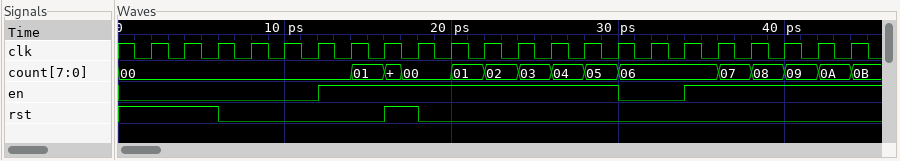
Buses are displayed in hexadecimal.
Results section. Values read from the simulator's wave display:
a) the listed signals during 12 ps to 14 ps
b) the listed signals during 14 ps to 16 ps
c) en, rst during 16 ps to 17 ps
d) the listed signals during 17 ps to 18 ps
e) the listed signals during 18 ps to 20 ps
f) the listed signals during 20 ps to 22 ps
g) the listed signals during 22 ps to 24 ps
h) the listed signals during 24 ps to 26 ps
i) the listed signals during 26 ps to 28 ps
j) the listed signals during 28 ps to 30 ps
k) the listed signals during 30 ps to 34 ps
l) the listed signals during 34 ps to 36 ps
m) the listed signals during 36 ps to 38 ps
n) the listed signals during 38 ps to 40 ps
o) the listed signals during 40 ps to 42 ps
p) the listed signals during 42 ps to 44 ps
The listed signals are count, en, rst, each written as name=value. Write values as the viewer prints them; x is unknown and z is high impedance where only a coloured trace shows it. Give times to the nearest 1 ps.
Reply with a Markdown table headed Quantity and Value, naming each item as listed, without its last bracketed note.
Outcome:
| Quantity | Value |
|---|---|
| the listed signals during 12 ps to 14 ps | count=00, en=1, rst=0 |
| the listed signals during 14 ps to 16 ps | count=01, en=1, rst=0 |
| en, rst during 16 ps to 17 ps | en=1, rst=1 |
| the listed signals during 17 ps to 18 ps | count=00, en=1, rst=1 |
| the listed signals during 18 ps to 20 ps | count=00, en=1, rst=0 |
| the listed signals during 20 ps to 22 ps | count=01, en=1, rst=0 |
| the listed signals during 22 ps to 24 ps | count=02, en=1, rst=0 |
| the listed signals during 24 ps to 26 ps | count=03, en=1, rst=0 |
| the listed signals during 26 ps to 28 ps | count=04, en=1, rst=0 |
| the listed signals during 28 ps to 30 ps | count=05, en=1, rst=0 |
| the listed signals during 30 ps to 34 ps | count=06, en=0, rst=0 |
| the listed signals during 34 ps to 36 ps | count=06, en=1, rst=0 |
| the listed signals during 36 ps to 38 ps | count=07, en=1, rst=0 |
| the listed signals during 38 ps to 40 ps | count=08, en=1, rst=0 |
| the listed signals during 40 ps to 42 ps | count=09, en=1, rst=0 |
| the listed signals during 42 ps to 44 ps | count=0A, en=1, rst=0 |
